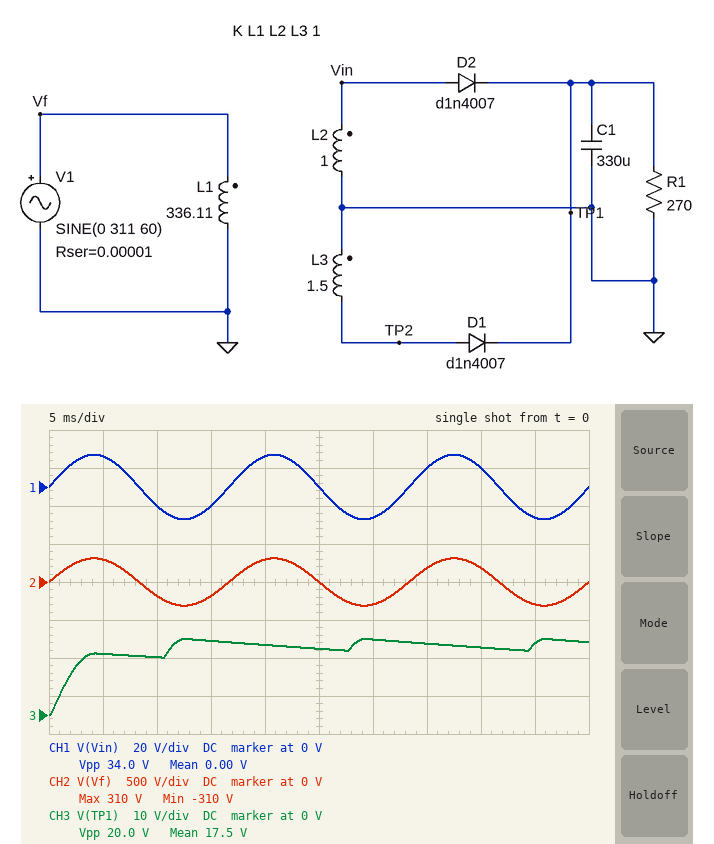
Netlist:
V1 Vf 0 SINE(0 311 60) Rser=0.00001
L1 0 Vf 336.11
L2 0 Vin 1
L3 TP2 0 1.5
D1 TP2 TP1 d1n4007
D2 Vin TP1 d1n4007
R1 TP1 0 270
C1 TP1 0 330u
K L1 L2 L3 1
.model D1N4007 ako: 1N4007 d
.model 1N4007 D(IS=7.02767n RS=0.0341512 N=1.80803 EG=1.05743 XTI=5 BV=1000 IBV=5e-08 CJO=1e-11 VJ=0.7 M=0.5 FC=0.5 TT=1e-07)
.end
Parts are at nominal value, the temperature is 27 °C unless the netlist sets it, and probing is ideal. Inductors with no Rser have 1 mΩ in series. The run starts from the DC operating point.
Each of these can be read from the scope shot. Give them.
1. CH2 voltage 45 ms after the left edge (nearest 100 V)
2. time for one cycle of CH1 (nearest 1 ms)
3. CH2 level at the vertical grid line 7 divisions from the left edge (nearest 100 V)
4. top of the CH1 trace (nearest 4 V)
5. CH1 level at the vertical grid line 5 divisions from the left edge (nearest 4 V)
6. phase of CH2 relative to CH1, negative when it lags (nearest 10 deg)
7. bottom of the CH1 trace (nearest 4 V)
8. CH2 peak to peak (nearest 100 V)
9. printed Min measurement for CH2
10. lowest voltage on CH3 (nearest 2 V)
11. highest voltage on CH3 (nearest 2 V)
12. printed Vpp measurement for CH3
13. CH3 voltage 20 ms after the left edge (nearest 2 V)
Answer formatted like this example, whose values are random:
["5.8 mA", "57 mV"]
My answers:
["-300 V", "17 ms", "200 V", "16 V", "0 V", "0 deg", "-16 V", "600 V", "-310 V", "0 V", "20 V", "20.0 V", "18 V"]
